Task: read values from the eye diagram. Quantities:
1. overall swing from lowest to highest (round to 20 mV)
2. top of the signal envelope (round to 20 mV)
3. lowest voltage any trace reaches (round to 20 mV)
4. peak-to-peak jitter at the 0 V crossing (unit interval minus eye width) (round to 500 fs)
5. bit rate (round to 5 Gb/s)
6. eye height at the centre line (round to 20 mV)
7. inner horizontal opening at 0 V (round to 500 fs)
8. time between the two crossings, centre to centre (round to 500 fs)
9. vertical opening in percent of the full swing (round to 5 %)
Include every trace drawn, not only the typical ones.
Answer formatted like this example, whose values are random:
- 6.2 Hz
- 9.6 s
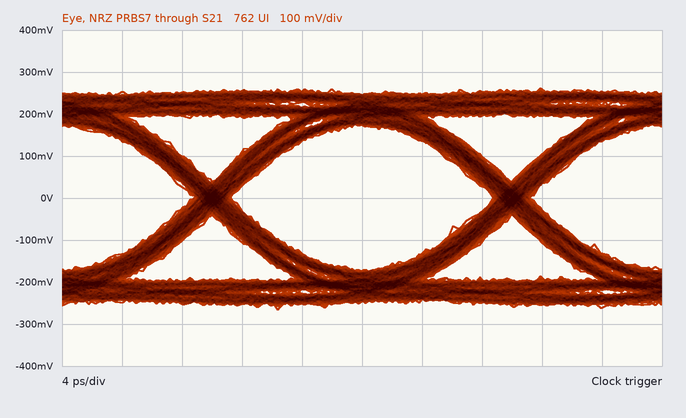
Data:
- 520 mV
- 260 mV
- -260 mV
- 2.5 ps
- 50 Gb/s
- 340 mV
- 17.5 ps
- 20.0 ps
- 65 %
